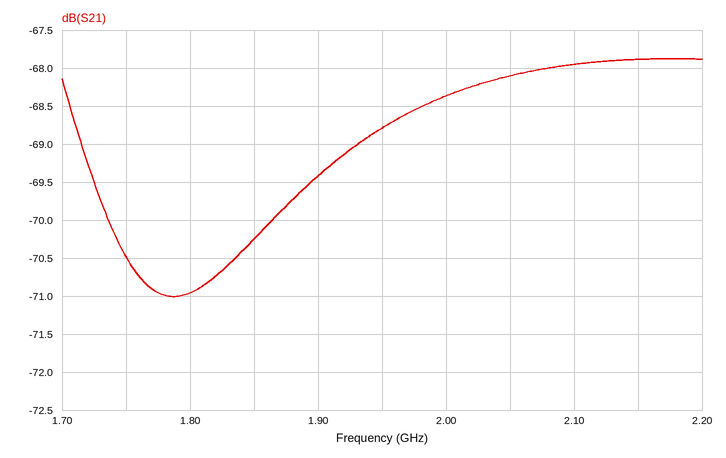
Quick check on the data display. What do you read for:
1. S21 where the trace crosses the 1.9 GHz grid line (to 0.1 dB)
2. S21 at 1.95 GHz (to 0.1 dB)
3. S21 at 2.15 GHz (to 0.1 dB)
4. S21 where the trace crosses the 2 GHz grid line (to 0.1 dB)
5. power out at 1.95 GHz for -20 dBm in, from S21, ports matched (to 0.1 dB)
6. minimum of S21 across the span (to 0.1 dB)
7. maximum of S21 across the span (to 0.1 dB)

-69.4 dB
-68.8 dB
-67.9 dB
-68.4 dB
-88.8 dBm
-71.0 dB
-67.9 dB
